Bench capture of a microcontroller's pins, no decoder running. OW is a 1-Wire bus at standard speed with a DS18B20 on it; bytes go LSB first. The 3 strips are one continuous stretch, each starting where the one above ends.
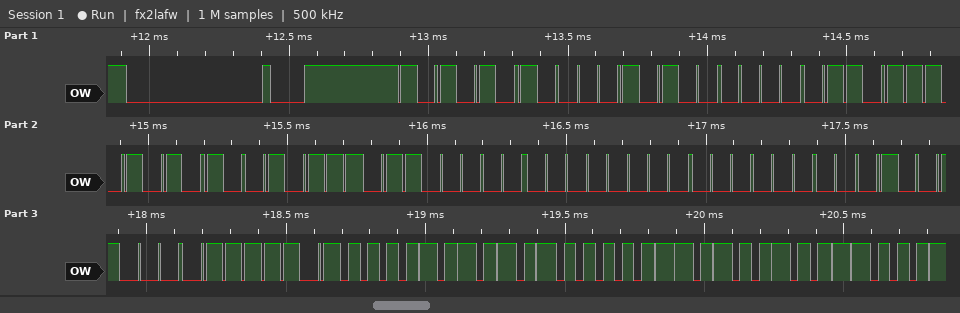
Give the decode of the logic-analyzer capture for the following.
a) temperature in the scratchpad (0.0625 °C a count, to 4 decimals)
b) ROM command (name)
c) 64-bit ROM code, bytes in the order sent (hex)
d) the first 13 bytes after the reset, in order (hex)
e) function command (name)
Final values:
85.0000 °C
Match ROM
28 60 57 E9 06 00 00 12
55 28 60 57 E9 06 00 00 12 BE 50 05 4B
Read Scratchpad
